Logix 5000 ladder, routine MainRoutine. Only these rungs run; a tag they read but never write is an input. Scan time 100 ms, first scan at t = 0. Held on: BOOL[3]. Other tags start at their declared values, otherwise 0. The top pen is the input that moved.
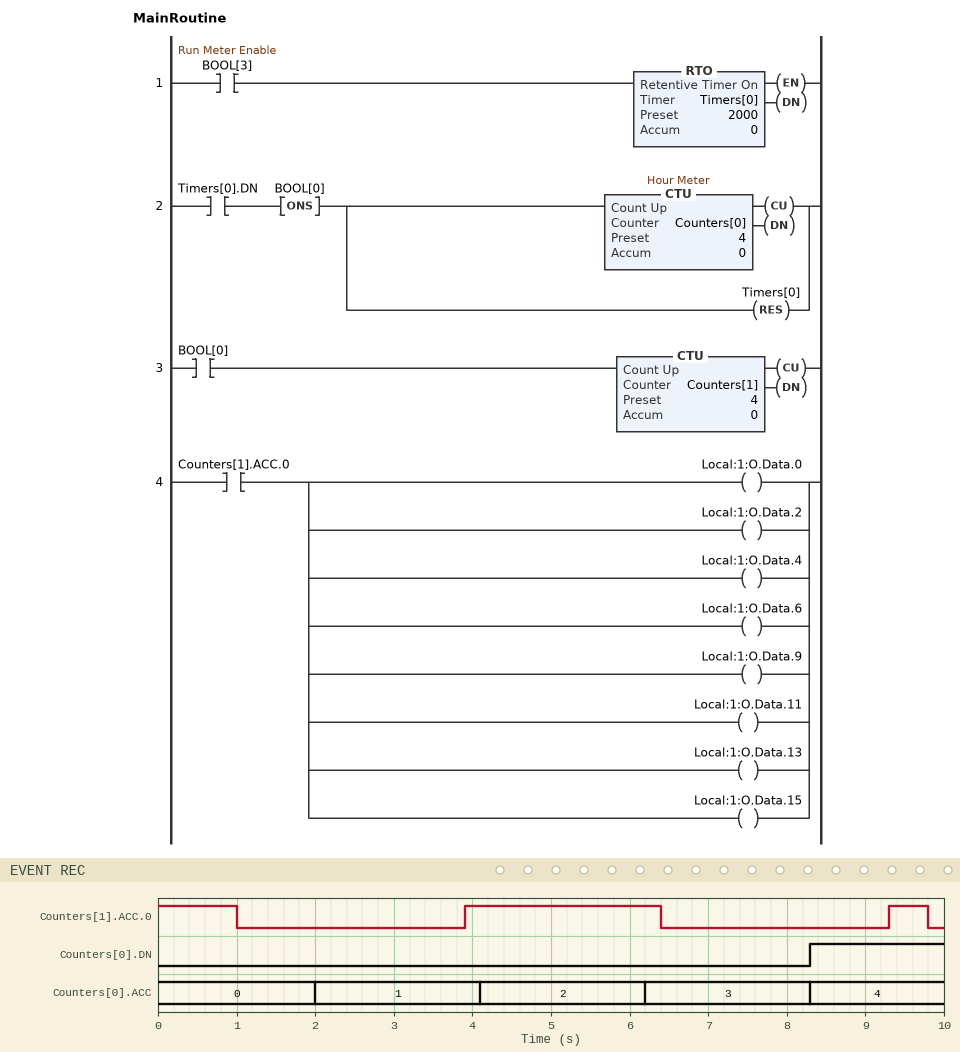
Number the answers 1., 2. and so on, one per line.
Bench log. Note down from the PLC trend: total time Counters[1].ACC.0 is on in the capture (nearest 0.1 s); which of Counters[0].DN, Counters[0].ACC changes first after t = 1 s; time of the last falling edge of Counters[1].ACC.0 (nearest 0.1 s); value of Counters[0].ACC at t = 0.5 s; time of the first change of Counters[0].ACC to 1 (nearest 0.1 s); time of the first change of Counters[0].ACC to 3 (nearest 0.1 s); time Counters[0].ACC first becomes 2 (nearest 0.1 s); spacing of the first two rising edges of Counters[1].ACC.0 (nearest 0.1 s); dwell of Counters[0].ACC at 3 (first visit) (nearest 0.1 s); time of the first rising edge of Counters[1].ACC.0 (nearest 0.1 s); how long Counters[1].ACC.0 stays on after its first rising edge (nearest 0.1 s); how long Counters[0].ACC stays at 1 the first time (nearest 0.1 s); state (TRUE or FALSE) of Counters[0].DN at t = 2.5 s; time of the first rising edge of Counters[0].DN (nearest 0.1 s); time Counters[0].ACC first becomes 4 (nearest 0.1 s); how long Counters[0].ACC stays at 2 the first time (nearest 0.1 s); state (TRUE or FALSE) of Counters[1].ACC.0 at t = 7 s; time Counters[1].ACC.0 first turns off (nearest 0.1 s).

1. 4.0 s
2. Counters[0].ACC
3. 9.8 s
4. 0
5. 2.0 s
6. 6.2 s
7. 4.1 s
8. 5.4 s
9. 2.1 s
10. 3.9 s
11. 2.5 s
12. 2.1 s
13. FALSE
14. 8.3 s
15. 8.3 s
16. 2.1 s
17. FALSE
18. 1.0 s
